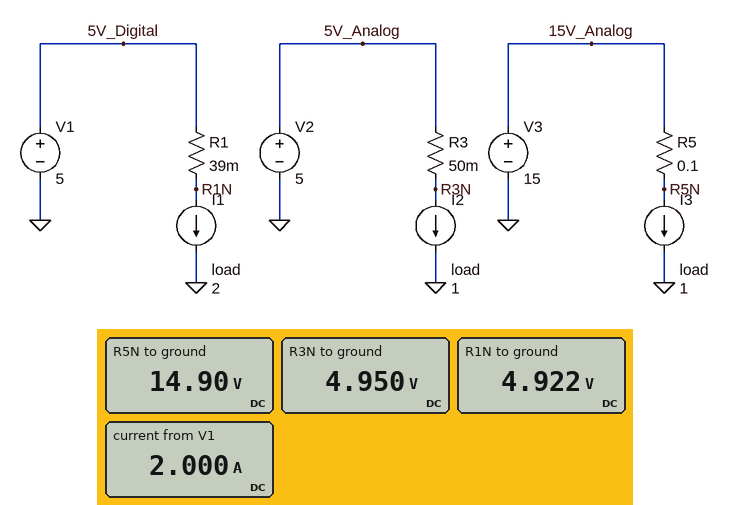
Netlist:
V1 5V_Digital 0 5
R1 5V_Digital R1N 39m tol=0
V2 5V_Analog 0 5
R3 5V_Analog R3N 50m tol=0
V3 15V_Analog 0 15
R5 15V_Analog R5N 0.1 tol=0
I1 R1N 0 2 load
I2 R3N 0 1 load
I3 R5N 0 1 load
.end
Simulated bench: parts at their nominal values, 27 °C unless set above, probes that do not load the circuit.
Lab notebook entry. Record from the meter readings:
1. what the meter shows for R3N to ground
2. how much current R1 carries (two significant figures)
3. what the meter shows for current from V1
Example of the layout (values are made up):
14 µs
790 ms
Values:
4.950 V
2.0 A
2.000 A
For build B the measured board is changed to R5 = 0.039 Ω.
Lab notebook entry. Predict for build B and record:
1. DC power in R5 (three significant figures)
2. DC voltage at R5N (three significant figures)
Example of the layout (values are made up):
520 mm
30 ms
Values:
39.0 mW
15.0 V
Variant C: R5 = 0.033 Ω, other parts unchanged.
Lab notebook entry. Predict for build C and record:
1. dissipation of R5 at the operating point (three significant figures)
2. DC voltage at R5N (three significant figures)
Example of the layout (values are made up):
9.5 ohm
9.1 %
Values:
33.0 mW
15.0 V
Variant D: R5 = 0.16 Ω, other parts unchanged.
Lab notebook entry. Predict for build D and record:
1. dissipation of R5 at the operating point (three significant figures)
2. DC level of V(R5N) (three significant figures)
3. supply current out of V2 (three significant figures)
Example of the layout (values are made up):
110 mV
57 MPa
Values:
160 mW
14.8 V
1.00 A
